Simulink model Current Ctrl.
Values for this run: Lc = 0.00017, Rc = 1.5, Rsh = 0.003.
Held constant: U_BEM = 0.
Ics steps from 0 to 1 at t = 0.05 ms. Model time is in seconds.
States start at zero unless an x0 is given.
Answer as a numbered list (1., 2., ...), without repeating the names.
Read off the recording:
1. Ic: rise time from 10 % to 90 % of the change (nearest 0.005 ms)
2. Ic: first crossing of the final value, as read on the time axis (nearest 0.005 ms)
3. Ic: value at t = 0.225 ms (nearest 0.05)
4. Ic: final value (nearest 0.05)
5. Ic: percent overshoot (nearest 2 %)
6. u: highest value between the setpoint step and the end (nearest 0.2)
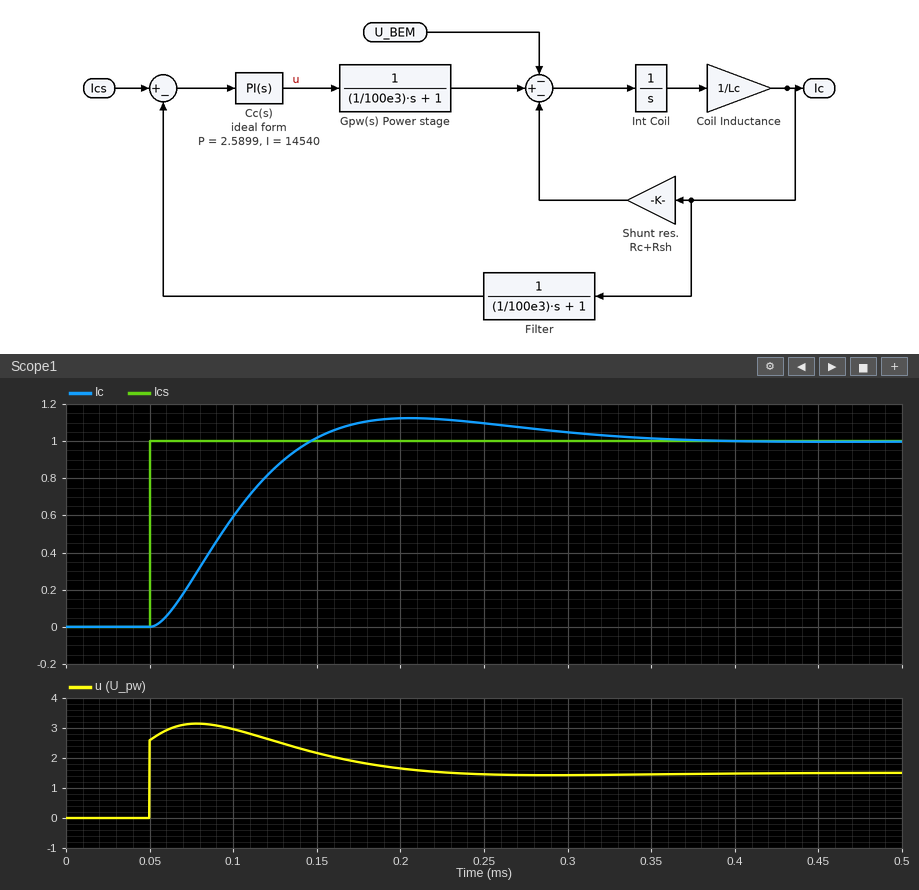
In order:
1. 0.065 ms
2. 0.145 ms
3. 1.10
4. 1.00
5. 12 %
6. 3.2
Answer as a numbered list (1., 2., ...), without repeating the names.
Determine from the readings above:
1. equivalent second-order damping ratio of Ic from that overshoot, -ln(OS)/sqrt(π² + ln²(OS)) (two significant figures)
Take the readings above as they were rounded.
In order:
1. 0.56
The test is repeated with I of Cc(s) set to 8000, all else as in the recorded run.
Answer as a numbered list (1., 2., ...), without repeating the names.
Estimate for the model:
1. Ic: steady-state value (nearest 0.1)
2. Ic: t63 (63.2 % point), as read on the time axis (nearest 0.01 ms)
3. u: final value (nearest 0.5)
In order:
1. 1.0
2. 0.11 ms
3. 1.5
